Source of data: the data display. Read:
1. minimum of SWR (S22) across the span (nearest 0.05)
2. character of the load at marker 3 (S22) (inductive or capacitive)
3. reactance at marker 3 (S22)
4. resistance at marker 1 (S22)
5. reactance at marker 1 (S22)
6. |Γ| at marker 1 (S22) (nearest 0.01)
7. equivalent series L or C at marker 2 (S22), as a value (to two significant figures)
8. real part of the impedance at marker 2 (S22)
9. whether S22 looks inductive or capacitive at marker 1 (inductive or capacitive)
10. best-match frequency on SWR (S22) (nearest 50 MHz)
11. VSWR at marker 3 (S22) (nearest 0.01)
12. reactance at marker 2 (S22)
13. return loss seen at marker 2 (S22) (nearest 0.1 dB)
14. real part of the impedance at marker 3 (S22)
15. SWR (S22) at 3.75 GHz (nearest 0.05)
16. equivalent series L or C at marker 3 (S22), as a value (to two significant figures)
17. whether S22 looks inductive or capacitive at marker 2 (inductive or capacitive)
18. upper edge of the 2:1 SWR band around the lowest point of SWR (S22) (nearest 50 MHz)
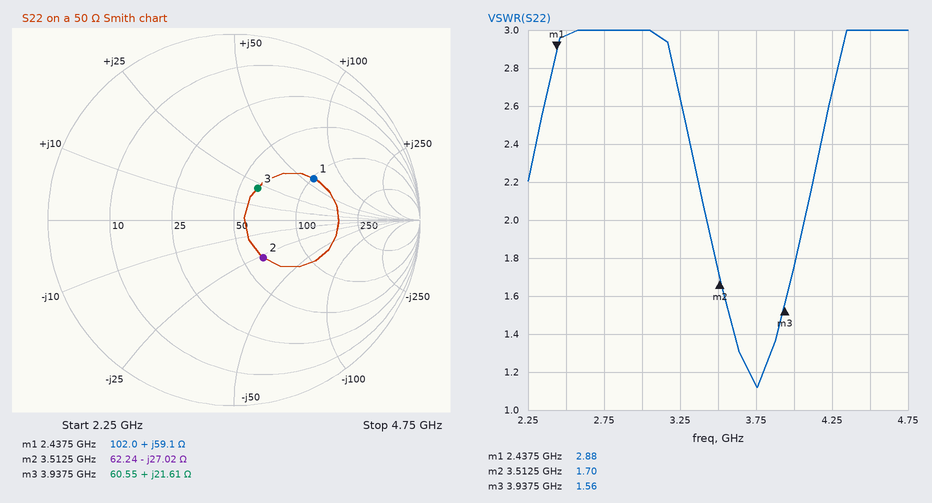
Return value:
1.10
inductive
+21.61 Ω
102.0 Ω
+59.1 Ω
0.48
1.7 pF
62.24 Ω
inductive
3.75 GHz
1.54
-27.02 Ω
11.8 dB
60.55 Ω
1.15
870 pH
capacitive
4.05 GHz
